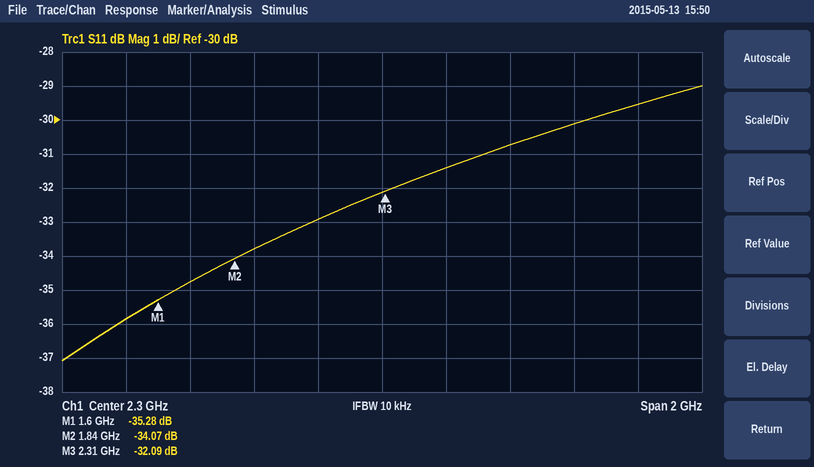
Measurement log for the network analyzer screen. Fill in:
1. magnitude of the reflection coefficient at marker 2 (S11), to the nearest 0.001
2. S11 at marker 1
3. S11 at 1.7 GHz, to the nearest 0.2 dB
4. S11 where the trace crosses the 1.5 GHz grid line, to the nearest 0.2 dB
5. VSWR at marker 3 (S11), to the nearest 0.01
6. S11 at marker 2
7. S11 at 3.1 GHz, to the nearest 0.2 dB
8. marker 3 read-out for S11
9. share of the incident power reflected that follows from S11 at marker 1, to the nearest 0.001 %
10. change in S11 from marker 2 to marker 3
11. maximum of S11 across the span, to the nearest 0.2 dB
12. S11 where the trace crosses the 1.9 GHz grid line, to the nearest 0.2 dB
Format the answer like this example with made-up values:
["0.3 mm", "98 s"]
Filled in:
["0.020", "-35.28 dB", "-34.8 dB", "-35.8 dB", "1.05", "-34.07 dB", "-29.6 dB", "-32.09 dB", "0.030 %", "1.98 dB", "-29.0 dB", "-33.8 dB"]
